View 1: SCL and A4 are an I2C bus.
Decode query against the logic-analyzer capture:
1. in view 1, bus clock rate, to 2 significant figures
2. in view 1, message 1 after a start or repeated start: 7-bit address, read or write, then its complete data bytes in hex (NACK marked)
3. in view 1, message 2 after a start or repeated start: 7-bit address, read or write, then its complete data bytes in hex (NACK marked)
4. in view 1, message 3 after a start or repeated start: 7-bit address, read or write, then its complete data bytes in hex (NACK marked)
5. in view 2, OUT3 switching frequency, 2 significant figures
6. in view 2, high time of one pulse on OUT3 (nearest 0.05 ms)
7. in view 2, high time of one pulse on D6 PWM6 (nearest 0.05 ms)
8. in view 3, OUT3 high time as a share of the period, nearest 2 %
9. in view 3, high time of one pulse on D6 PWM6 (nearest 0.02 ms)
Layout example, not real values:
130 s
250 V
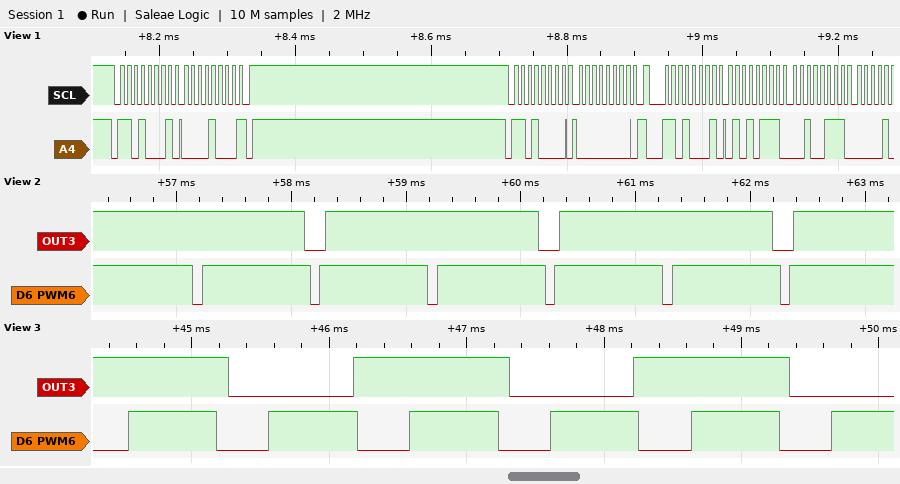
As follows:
100 kHz
0x68 read: 08 NACK
0x68 write: 00
0x68 read: 57 27
490 Hz
1.85 ms
0.95 ms
56 %
0.64 ms
